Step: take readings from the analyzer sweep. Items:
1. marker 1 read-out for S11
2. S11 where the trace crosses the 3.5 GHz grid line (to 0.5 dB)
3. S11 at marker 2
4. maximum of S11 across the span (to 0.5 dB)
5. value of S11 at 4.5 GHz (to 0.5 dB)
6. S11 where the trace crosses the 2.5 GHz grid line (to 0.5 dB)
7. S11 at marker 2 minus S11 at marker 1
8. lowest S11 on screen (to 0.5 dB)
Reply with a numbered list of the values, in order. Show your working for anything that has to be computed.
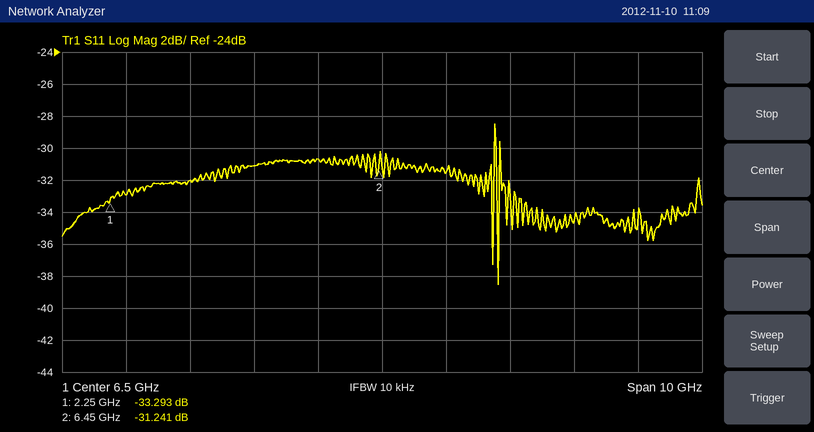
1. -33.293 dB
2. -32.0 dB
3. -31.241 dB
4. -28.5 dB
5. -31.0 dB
6. -33.0 dB
7. -31.241 − (-33.293) = 2.052 dB
8. -38.5 dB
